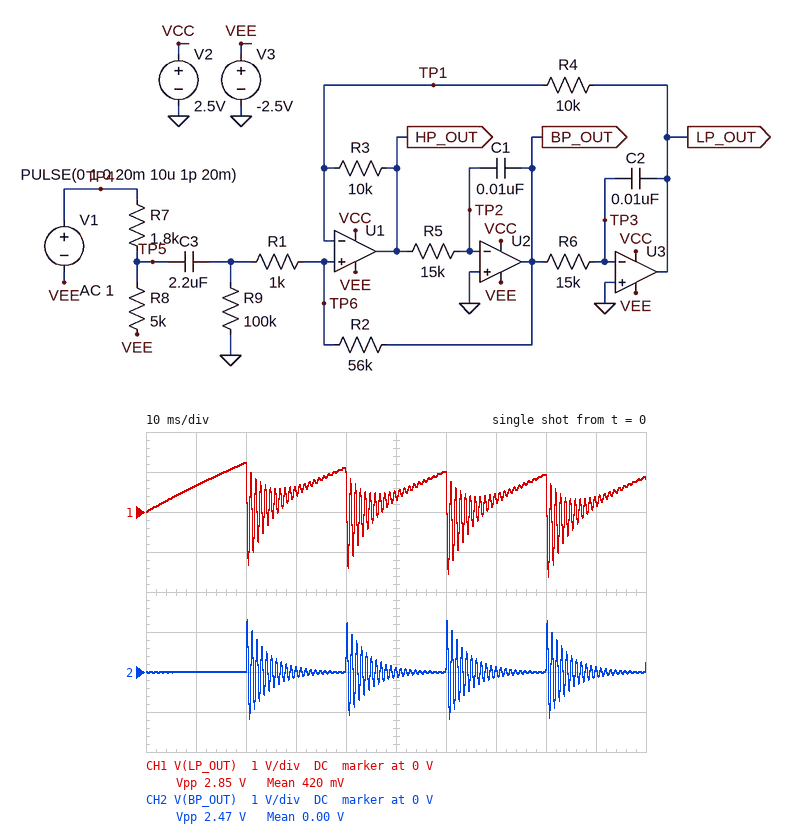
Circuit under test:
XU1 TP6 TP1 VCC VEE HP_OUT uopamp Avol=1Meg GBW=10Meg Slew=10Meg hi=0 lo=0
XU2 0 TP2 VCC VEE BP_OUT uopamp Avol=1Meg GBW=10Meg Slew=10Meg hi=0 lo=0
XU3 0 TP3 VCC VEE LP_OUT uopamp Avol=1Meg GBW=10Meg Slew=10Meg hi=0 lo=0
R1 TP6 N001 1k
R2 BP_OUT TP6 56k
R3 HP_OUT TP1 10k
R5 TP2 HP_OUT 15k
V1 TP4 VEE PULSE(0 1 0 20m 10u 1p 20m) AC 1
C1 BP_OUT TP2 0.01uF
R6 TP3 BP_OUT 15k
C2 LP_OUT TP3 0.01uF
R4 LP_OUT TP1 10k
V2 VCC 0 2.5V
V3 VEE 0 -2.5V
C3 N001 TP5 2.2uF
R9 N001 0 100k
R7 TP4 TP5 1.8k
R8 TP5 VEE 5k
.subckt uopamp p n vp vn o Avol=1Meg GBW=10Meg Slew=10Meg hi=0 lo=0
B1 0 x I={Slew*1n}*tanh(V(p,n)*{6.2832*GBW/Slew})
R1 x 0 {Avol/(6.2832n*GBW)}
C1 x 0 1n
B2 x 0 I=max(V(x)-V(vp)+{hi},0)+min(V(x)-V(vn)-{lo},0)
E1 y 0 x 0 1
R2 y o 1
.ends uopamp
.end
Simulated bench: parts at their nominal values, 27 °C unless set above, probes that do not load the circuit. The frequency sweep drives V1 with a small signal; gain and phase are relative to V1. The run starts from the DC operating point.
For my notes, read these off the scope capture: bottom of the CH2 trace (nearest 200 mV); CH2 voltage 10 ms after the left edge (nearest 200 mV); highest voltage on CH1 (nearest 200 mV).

-1.2 V
0 V
1.2 V
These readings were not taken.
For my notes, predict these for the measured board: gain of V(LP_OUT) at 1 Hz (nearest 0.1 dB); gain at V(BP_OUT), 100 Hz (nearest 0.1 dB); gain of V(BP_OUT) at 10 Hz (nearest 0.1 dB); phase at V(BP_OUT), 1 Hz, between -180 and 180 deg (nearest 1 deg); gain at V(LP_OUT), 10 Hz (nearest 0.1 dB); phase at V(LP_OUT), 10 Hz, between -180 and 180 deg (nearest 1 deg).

-3.8 dB
-17.6 dB
-37.8 dB
-28 deg
2.7 dB
11 deg
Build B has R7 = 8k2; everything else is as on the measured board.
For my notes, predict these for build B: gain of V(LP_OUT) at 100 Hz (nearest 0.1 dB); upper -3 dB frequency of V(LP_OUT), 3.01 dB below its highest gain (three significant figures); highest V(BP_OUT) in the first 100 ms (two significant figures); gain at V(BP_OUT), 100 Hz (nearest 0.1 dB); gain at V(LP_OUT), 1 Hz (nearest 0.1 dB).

-3.2 dB
1.13 kHz
610 mV
-23.7 dB
-9.7 dB
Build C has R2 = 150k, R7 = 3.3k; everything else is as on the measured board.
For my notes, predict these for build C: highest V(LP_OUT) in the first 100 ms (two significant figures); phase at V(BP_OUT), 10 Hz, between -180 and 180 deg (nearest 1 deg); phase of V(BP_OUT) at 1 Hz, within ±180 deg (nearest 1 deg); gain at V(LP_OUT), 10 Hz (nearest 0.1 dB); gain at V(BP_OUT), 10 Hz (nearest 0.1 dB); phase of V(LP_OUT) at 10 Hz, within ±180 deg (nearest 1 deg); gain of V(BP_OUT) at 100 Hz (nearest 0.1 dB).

1.1 V
-83 deg
-41 deg
1.2 dB
-39.3 dB
7 deg
-19.2 dB
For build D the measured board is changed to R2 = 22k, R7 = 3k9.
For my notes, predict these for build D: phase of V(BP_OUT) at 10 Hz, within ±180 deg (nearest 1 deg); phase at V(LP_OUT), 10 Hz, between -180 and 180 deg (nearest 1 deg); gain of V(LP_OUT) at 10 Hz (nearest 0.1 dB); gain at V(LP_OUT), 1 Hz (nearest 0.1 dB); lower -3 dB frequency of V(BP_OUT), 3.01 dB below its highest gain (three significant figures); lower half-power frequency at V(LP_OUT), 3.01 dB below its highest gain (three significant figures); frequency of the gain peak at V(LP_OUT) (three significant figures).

-71 deg
19 deg
-0.9 dB
-11.5 dB
939 Hz
903 Hz
1.05 kHz
